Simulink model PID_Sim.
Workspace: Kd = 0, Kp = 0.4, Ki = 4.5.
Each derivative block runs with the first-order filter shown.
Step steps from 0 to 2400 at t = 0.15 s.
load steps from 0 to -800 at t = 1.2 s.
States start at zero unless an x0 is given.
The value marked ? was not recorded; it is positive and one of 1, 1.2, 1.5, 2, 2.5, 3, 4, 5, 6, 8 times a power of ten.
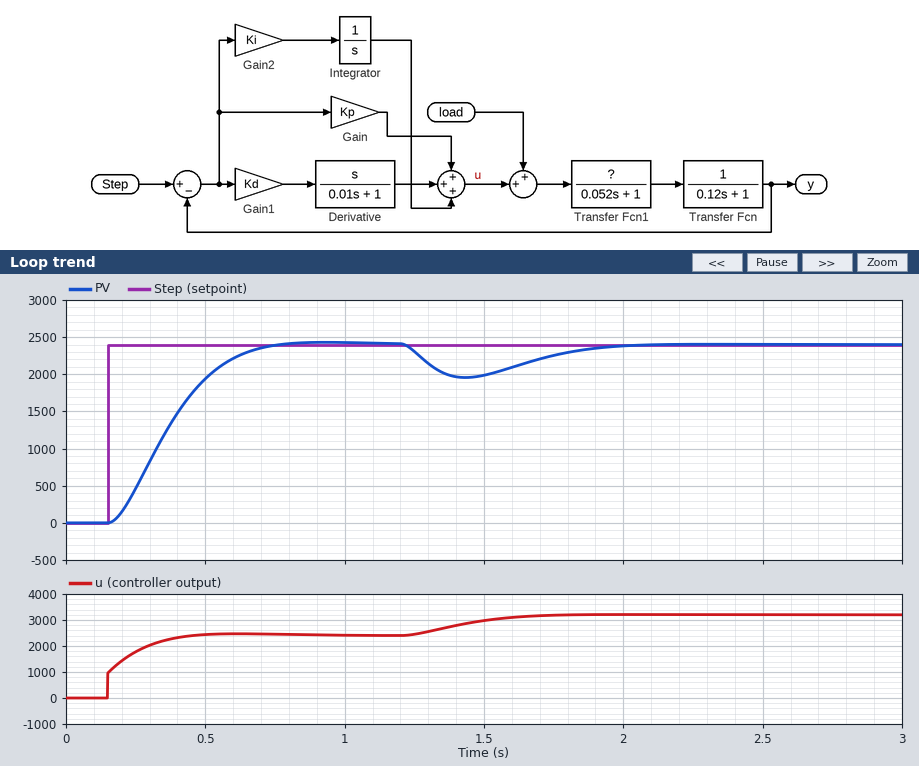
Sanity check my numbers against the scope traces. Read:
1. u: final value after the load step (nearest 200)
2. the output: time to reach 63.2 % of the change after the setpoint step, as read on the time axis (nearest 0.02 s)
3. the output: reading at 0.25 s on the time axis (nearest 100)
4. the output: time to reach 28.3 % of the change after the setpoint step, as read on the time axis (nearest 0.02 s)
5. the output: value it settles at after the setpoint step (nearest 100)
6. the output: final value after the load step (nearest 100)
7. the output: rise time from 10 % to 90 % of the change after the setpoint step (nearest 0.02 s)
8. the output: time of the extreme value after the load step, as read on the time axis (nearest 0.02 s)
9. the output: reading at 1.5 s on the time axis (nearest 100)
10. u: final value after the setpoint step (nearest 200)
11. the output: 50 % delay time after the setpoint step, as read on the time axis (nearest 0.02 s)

3200
0.40 s
500
0.28 s
2400
2400
0.36 s
1.44 s
2000
2400
0.36 s
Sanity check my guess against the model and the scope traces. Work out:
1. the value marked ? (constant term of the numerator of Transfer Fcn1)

1
